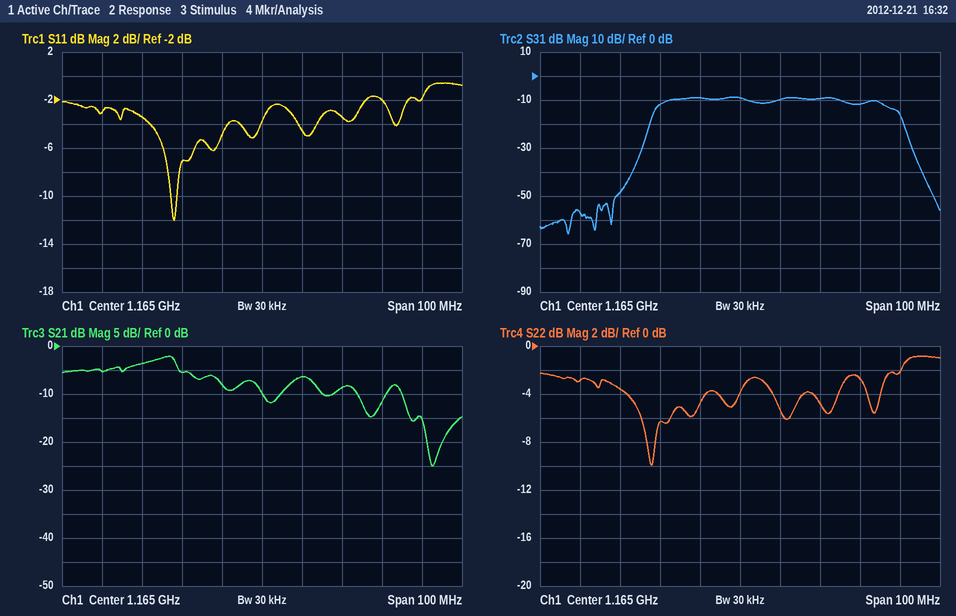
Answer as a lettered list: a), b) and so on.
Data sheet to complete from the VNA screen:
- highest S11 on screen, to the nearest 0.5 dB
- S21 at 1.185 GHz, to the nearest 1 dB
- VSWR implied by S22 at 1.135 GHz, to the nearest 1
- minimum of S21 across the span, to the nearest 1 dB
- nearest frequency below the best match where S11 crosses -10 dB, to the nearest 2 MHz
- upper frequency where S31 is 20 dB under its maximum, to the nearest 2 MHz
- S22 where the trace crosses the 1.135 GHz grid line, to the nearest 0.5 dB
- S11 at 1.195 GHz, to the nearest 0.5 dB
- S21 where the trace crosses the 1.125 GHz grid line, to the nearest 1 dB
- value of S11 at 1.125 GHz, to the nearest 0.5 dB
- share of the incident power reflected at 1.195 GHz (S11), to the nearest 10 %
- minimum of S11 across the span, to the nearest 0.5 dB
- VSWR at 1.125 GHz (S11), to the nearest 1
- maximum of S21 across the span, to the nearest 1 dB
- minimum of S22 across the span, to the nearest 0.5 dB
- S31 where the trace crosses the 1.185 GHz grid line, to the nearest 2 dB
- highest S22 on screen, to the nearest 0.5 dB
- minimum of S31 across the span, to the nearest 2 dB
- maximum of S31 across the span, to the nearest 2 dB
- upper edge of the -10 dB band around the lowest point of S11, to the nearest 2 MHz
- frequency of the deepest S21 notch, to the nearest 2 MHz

a) -0.5 dB
b) -9 dB
c) 5
d) -25 dB
e) 1.142 GHz
f) 1.208 GHz
g) -3.5 dB
h) -2.0 dB
i) -5 dB
j) -3.0 dB
k) 60 %
l) -12.0 dB
m) 6
n) -2 dB
o) -10.0 dB
p) -10 dB
q) -1.0 dB
r) -66 dB
s) -8 dB
t) 1.144 GHz
u) 1.208 GHz
